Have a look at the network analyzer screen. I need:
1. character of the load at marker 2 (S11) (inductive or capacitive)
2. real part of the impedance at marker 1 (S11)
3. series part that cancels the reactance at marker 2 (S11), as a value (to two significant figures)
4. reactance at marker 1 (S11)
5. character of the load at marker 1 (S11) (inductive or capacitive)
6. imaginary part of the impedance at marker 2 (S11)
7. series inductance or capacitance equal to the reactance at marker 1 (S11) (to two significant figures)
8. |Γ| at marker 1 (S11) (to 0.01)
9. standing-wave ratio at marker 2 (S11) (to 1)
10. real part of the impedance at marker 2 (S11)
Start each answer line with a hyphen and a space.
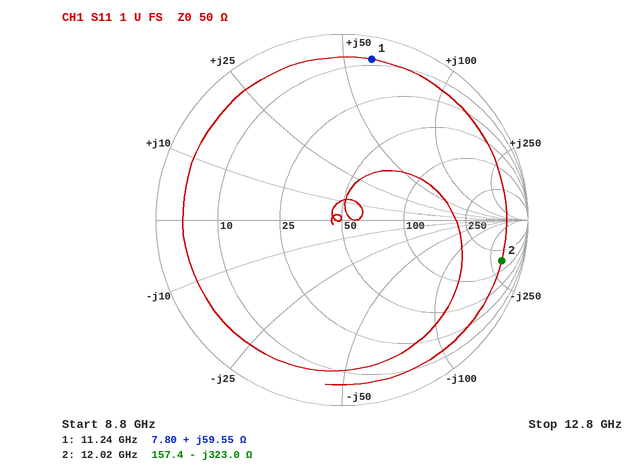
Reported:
- capacitive
- 7.80 Ω
- 4.3 nH
- +59.55 Ω
- inductive
- -323.0 Ω
- 840 pH
- 0.88
- 17
- 157.4 Ω
